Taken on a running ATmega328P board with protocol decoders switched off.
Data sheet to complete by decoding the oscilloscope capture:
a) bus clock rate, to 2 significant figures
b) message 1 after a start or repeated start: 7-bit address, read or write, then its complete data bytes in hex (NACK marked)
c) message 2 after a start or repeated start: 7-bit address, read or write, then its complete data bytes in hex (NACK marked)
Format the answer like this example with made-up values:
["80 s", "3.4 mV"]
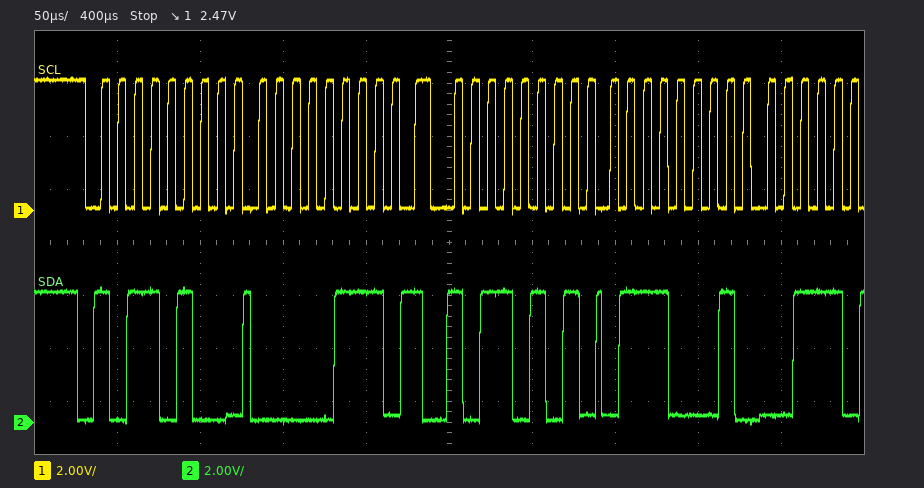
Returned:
["100 kHz", "0x5A write: 07", "0x5A read: 71"]
